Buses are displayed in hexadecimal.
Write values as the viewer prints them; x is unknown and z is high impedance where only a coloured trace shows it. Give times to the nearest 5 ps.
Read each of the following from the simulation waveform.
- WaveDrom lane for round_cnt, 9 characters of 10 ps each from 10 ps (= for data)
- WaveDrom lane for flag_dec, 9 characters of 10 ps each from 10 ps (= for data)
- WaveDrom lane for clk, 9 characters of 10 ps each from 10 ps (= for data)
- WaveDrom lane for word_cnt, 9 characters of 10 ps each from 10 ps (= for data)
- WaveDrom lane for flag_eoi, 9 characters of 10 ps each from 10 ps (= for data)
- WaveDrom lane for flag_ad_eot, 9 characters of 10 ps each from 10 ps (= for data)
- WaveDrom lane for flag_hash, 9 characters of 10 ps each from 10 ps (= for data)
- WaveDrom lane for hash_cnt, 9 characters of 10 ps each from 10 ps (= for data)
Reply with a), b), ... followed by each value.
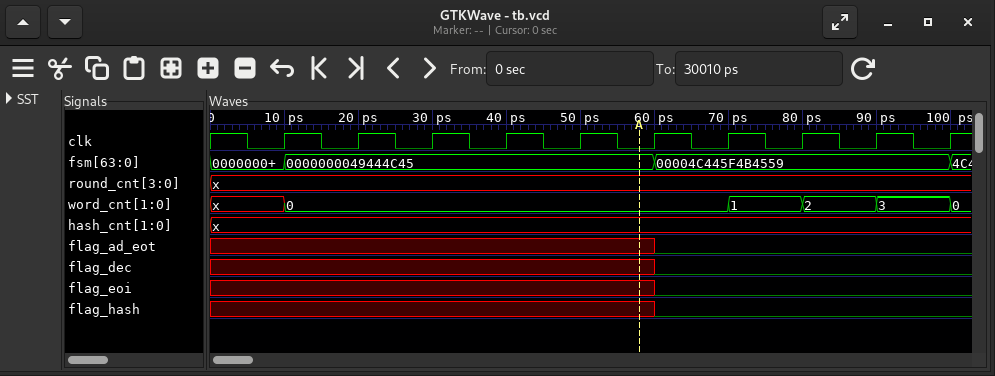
a) {name: 'round_cnt', wave: 'x........'}
b) {name: 'flag_dec', wave: 'x....0...'}
c) {name: 'clk', wave: 'p........'}
d) {name: 'word_cnt', wave: '=.....===', data: '0 1 2 3'}
e) {name: 'flag_eoi', wave: 'x....0...'}
f) {name: 'flag_ad_eot', wave: 'x....0...'}
g) {name: 'flag_hash', wave: 'x....0...'}
h) {name: 'hash_cnt', wave: 'x........'}
